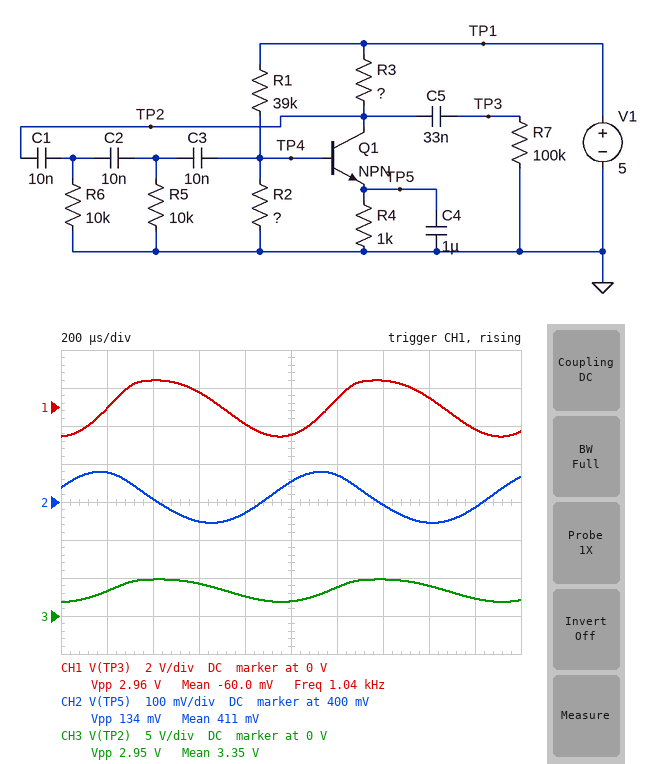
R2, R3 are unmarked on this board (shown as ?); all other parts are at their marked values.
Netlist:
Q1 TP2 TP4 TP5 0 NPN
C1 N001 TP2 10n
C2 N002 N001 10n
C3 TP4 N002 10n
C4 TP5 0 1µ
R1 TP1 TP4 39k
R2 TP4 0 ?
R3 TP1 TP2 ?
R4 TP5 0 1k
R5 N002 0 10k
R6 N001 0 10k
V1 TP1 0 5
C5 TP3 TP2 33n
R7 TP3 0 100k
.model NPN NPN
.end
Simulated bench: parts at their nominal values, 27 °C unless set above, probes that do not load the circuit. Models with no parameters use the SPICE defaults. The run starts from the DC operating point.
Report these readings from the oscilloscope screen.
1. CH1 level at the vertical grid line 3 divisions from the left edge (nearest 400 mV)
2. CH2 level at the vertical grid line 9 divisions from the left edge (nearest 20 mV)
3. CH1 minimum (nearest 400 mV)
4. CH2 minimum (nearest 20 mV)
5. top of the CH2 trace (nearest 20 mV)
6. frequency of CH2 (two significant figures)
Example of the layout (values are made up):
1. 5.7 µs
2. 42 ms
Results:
1. 800 mV
2. 380 mV
3. -1.6 V
4. 340 mV
5. 480 mV
6. 1.0 kHz
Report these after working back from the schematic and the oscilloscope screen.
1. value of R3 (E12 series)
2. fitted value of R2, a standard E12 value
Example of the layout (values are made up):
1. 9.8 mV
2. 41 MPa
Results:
1. 3.9 kΩ
2. 12 kΩ
